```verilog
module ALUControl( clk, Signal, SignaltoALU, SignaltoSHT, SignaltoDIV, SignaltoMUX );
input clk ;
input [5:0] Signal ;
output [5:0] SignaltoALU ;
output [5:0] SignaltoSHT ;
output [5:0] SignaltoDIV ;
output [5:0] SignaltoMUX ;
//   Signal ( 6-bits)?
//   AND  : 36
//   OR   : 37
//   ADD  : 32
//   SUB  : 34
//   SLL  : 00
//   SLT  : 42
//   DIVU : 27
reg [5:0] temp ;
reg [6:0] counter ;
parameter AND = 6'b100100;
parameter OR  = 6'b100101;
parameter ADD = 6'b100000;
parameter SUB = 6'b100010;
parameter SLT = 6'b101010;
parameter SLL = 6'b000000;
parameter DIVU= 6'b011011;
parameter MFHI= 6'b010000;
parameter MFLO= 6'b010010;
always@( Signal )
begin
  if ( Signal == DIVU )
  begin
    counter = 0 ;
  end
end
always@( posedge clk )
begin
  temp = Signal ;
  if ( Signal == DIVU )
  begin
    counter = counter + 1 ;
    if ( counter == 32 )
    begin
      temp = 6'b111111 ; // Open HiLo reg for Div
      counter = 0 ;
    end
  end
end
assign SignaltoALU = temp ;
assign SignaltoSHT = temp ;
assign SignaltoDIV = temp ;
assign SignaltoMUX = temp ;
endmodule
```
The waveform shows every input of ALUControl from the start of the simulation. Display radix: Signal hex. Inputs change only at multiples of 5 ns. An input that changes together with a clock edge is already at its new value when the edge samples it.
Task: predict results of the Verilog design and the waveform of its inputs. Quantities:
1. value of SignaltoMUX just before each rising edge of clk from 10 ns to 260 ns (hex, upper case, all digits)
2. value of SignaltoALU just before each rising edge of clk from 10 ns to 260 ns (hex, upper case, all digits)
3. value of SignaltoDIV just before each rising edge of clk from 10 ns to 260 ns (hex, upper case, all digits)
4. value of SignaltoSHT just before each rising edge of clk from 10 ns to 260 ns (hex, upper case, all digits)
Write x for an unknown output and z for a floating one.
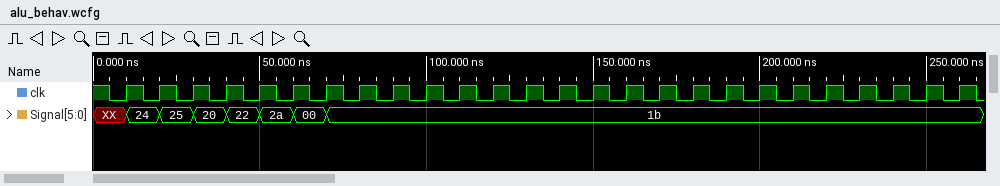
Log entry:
x, 24, 25, 20, 22, 2A, 00, 1B, 1B, 1B, 1B, 1B, 1B, 1B, 1B, 1B, 1B, 1B, 1B, 1B, 1B, 1B, 1B, 1B, 1B, 1B
x, 24, 25, 20, 22, 2A, 00, 1B, 1B, 1B, 1B, 1B, 1B, 1B, 1B, 1B, 1B, 1B, 1B, 1B, 1B, 1B, 1B, 1B, 1B, 1B
x, 24, 25, 20, 22, 2A, 00, 1B, 1B, 1B, 1B, 1B, 1B, 1B, 1B, 1B, 1B, 1B, 1B, 1B, 1B, 1B, 1B, 1B, 1B, 1B
x, 24, 25, 20, 22, 2A, 00, 1B, 1B, 1B, 1B, 1B, 1B, 1B, 1B, 1B, 1B, 1B, 1B, 1B, 1B, 1B, 1B, 1B, 1B, 1B
